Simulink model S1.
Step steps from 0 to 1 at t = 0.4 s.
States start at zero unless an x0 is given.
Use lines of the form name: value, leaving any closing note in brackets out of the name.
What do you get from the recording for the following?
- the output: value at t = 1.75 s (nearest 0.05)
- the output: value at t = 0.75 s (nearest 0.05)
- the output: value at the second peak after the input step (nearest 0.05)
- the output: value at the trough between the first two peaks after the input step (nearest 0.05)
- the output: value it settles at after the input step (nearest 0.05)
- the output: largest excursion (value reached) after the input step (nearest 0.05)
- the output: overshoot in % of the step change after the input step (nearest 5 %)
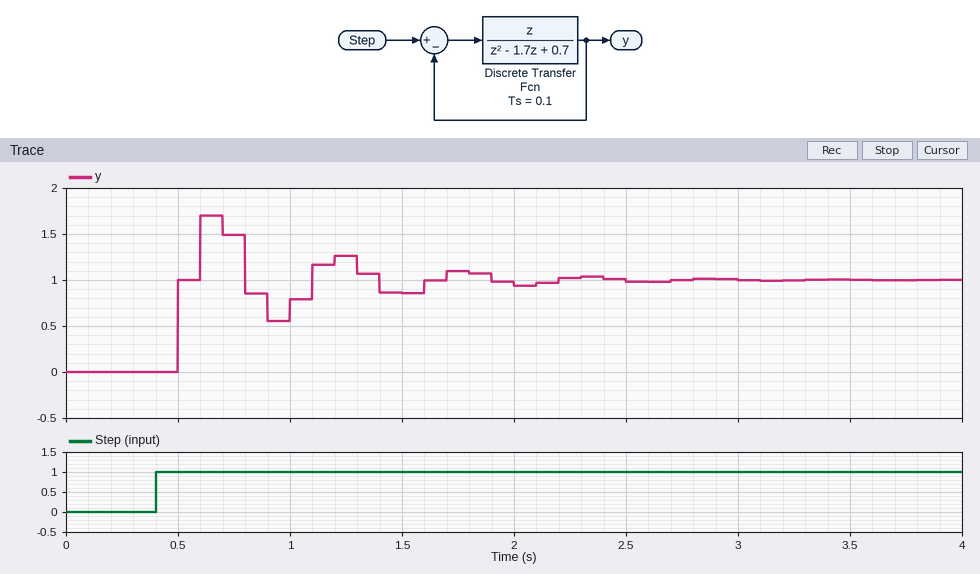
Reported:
the output: value at t = 1.75 s: 1.10
the output: value at t = 0.75 s: 1.50
the output: value at the second peak after the input step: 1.25
the output: value at the trough between the first two peaks after the input step: 0.55
the output: value it settles at after the input step: 1.00
the output: largest excursion (value reached) after the input step: 1.70
the output: overshoot in % of the step change after the input step: 70 %
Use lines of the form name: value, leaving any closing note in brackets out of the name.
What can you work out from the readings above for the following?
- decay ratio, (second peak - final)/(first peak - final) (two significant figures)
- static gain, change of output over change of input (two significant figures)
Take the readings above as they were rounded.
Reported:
decay ratio, (second peak - final)/(first peak - final): 0.36
static gain, change of output over change of input: 1.0
